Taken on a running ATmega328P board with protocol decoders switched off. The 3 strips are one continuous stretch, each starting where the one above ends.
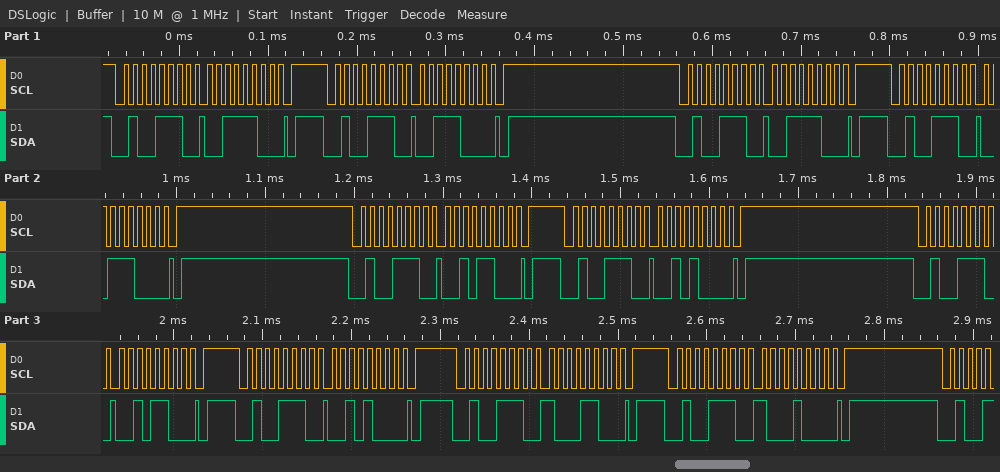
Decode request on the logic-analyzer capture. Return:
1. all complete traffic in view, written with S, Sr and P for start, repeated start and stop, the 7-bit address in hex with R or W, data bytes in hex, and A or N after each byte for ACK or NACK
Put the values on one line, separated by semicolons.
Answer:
S 27W A 3C A P S 27W A 38 A P S 27W A 3C A P S 27W A 38 A P S 27W A 2C A P S 27W A 28 A P S 27W A 2C A P S 27W A 28 A P S 27W A 8C A P S 27W A 88 A P
